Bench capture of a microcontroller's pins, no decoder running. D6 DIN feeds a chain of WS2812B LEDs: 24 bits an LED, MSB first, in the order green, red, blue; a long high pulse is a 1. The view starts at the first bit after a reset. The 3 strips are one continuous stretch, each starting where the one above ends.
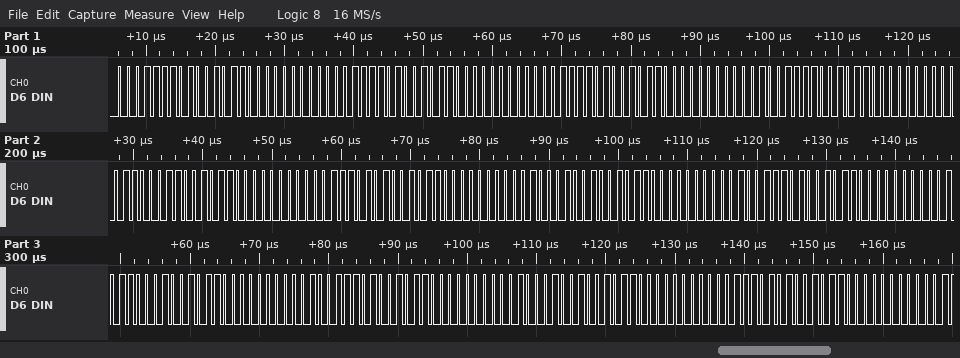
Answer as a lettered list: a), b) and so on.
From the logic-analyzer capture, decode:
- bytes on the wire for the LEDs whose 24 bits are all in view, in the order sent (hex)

a) 1E 96 00 1E 96 00 1E 96 00 27 96 00 31 96 00 3A 96 00 44 96 00 4E 96 00 58 96 00 4E 96 00 44 96 00 3A 96 00
